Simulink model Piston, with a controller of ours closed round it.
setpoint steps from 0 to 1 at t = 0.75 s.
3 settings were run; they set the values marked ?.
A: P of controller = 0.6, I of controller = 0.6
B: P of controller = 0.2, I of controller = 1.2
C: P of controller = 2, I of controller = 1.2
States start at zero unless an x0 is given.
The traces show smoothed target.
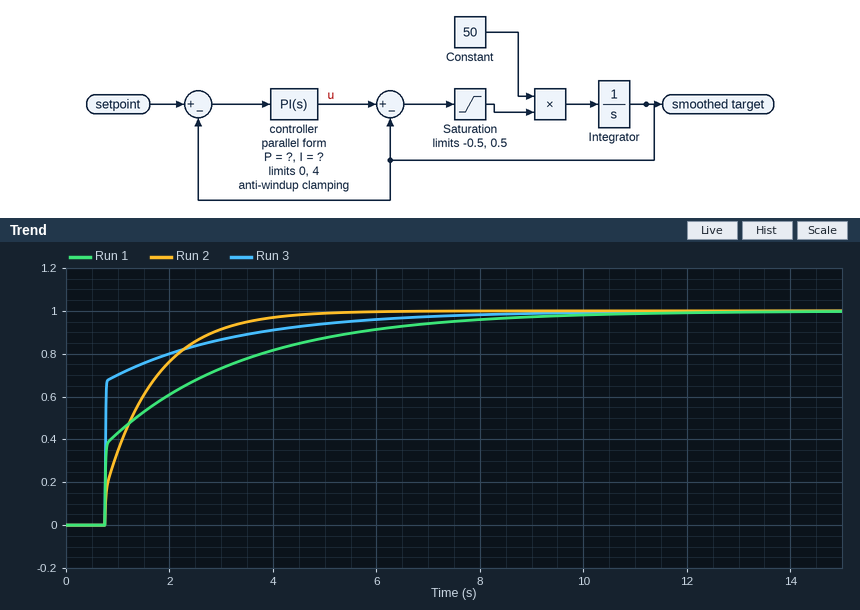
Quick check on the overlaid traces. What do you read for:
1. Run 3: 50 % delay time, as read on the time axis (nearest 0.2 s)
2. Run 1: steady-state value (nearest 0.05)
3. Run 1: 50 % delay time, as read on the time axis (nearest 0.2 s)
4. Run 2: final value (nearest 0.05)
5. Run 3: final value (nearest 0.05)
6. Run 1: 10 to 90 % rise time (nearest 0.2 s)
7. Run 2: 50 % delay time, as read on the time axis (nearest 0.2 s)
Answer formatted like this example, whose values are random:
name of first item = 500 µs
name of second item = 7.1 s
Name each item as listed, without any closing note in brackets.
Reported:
Run 3: 50 % delay time, as read on the time axis = 0.8 s
Run 1: steady-state value = 1.00
Run 1: 50 % delay time, as read on the time axis = 1.4 s
Run 2: final value = 1.00
Run 3: final value = 1.00
Run 1: 10 to 90 % rise time = 4.8 s
Run 2: 50 % delay time, as read on the time axis = 1.2 s
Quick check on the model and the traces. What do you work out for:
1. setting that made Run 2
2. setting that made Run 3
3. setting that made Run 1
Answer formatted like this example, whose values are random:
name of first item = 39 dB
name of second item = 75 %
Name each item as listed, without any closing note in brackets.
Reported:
setting that made Run 2 = B
setting that made Run 3 = C
setting that made Run 1 = A
